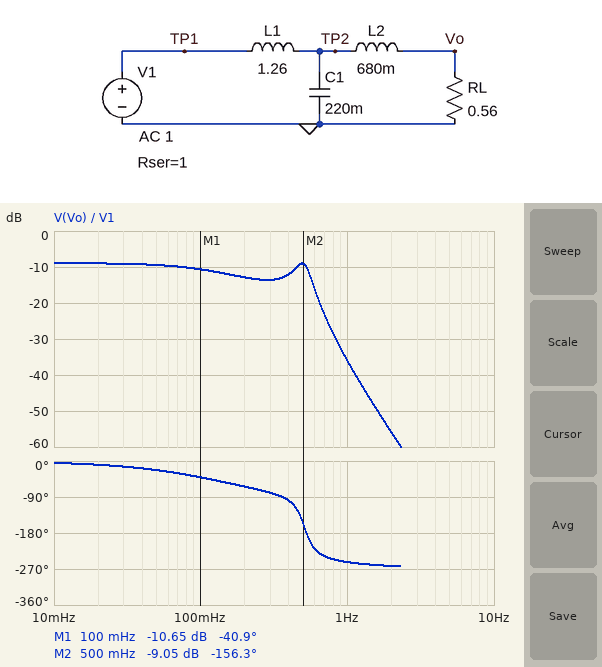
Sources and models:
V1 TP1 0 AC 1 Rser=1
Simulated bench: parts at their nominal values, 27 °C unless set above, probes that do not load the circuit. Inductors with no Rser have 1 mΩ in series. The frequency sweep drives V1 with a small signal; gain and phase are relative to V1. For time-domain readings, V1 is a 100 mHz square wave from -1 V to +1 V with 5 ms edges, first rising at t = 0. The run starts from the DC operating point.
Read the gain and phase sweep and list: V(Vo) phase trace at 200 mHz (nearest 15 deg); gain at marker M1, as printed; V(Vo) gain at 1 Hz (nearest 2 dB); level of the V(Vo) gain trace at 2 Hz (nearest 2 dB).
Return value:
-60 deg
-10.65 dB
-36 dB
-56 dB
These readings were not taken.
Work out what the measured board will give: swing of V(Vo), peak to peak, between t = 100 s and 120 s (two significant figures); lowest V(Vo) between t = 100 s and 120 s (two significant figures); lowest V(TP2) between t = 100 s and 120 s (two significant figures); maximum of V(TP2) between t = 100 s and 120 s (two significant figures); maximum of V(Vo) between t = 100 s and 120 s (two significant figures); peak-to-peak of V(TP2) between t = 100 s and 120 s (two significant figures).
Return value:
730 mV
-370 mV
-890 mV
890 mV
370 mV
1.8 V
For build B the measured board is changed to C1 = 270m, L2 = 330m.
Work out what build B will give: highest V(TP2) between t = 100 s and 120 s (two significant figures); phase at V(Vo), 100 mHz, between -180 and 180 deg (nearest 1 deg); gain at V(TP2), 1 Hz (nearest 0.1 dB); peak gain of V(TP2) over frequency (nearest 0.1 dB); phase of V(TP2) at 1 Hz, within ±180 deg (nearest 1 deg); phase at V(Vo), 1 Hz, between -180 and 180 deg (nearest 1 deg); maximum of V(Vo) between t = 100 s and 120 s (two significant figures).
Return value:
450 mV
-36 deg
-19.1 dB
-4.9 dB
-166 deg
119 deg
360 mV
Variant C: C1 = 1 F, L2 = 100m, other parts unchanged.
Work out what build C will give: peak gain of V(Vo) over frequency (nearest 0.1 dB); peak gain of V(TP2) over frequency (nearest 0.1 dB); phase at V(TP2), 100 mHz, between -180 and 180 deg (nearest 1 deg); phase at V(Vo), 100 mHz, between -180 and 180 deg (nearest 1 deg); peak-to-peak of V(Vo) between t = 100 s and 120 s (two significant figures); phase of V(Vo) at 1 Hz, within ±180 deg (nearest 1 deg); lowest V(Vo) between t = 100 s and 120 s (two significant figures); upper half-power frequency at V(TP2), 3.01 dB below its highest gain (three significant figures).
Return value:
-8.9 dB
-8.9 dB
-37 deg
-43 deg
720 mV
148 deg
-360 mV
213 mHz
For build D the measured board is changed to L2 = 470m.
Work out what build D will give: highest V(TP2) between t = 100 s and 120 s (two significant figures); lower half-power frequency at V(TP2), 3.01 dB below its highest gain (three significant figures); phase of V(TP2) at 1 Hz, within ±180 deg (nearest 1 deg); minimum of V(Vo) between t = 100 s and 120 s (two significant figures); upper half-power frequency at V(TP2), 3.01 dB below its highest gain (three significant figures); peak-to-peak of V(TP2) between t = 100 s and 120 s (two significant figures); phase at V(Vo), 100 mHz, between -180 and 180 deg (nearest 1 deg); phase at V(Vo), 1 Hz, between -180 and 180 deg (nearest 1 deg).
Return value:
610 mV
469 mHz
-168 deg
-360 mV
647 mHz
1.2 V
-38 deg
113 deg
